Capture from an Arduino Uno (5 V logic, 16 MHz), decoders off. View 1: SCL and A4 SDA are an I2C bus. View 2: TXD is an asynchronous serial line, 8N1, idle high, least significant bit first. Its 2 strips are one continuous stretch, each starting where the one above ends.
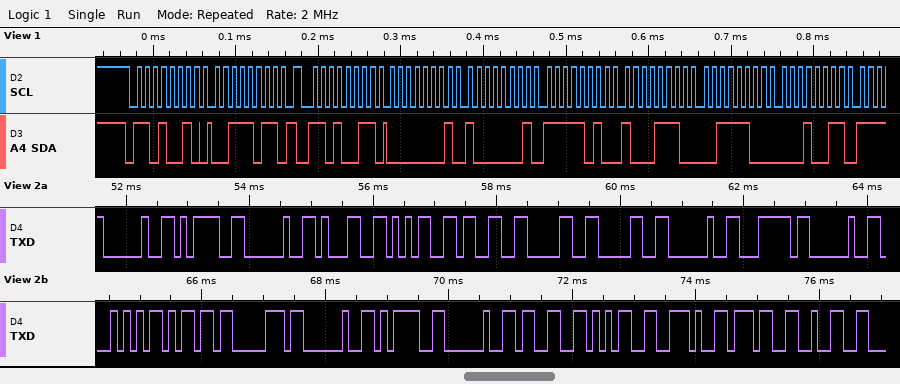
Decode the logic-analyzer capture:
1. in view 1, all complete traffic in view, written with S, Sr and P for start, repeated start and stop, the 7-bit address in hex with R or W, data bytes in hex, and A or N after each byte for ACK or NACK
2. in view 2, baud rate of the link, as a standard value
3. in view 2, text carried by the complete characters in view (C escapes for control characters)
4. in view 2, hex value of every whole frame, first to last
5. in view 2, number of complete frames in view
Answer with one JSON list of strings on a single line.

["S 69W A 3B A Sr 69R A 01 A 81 A FA A 8E A 3C A 13 A", "9600 baud", "\" = 15300 | Tmp = 35.72\"", "20 3D 20 31 35 33 30 30 20 7C 20 54 6D 70 20 3D 20 33 35 2E 37 32", "22"]
